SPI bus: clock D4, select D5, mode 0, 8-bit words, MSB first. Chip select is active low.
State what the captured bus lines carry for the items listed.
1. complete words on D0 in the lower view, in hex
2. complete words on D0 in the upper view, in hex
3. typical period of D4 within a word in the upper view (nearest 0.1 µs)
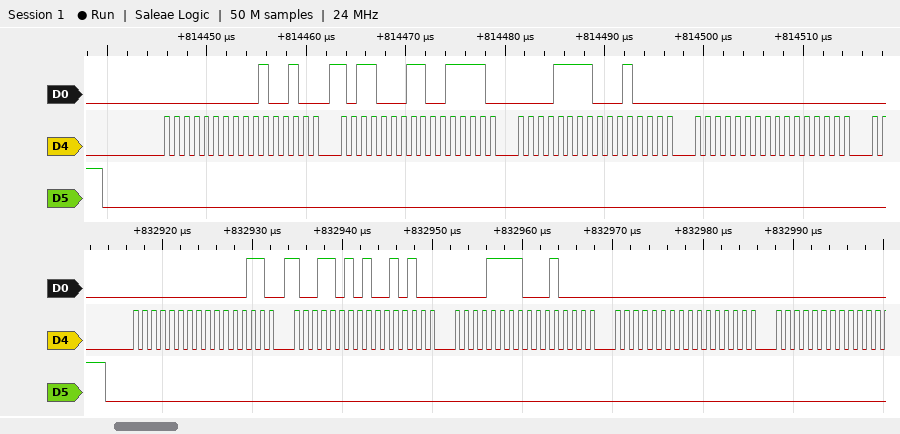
00, 06, 9A, 94, 0F, 10, 00, 00, 00
00, 24, B1, 9E, 0F, 10, 00, 00
1 µs
